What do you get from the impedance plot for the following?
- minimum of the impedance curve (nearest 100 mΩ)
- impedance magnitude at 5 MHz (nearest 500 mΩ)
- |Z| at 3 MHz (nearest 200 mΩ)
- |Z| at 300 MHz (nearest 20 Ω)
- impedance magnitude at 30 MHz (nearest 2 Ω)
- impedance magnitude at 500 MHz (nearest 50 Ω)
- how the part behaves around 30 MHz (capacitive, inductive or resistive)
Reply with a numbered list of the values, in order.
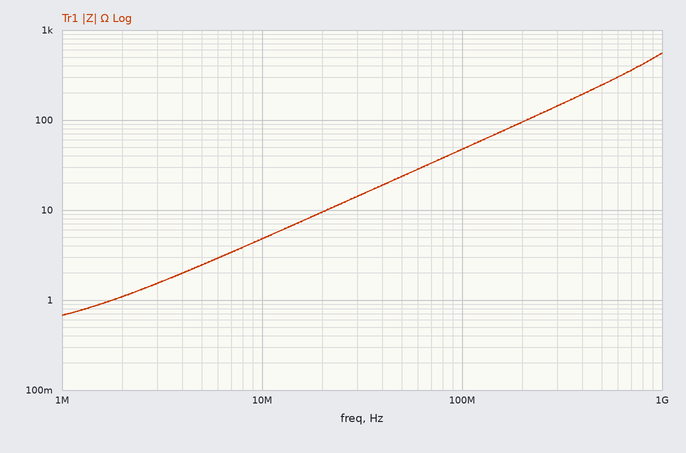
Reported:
1. 700 mΩ
2. 2.5 Ω
3. 1.6 Ω
4. 140 Ω
5. 14 Ω
6. 250 Ω
7. inductive
